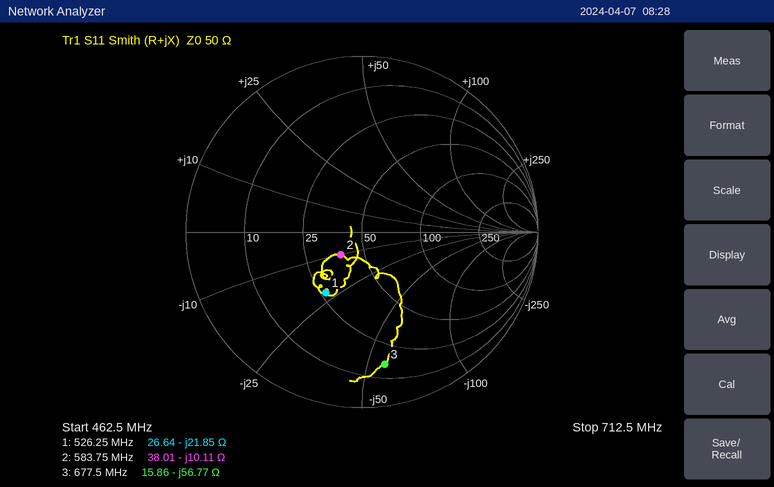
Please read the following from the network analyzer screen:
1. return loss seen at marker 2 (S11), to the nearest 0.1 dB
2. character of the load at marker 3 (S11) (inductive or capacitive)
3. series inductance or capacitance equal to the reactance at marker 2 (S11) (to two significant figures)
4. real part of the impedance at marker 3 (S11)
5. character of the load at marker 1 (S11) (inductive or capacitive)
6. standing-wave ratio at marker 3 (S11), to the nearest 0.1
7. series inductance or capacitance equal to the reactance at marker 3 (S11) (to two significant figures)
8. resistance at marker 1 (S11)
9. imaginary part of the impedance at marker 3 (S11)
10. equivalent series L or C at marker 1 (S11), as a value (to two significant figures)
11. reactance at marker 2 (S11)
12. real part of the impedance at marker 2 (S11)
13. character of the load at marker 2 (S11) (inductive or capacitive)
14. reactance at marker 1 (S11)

15.0 dB
capacitive
27 pF
15.86 Ω
capacitive
7.4
4.1 pF
26.64 Ω
-56.77 Ω
14 pF
-10.11 Ω
38.01 Ω
capacitive
-21.85 Ω
